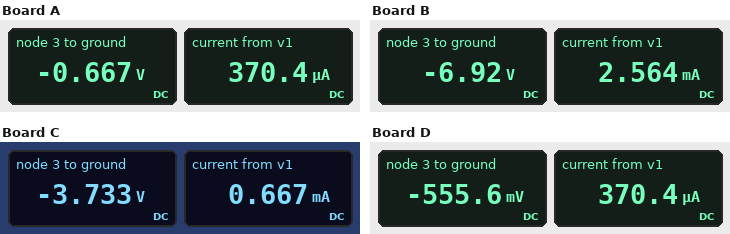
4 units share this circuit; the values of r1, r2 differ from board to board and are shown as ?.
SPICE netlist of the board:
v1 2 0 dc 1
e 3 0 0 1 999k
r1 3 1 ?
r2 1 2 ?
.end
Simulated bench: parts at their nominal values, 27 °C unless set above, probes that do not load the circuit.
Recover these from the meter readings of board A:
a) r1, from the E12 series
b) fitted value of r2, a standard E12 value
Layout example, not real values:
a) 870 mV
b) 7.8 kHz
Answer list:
a) 1.8 kΩ
b) 2.7 kΩ
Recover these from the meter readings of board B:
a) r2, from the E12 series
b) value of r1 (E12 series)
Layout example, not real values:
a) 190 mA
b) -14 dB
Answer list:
a) 390 Ω
b) 2.7 kΩ
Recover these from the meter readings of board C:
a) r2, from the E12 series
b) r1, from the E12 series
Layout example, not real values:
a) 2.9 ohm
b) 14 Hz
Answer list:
a) 1.5 kΩ
b) 5.6 kΩ
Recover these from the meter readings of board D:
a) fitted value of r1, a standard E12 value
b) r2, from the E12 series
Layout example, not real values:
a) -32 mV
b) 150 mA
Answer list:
a) 1.5 kΩ
b) 2.7 kΩ
